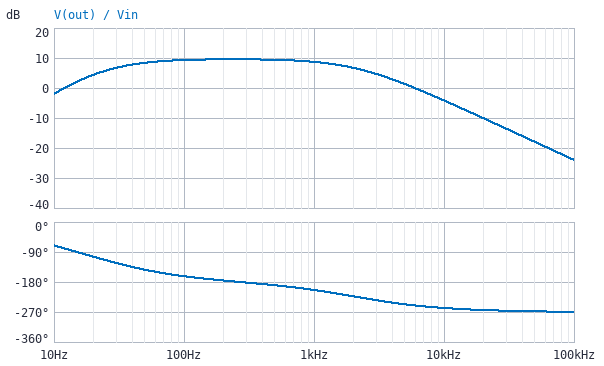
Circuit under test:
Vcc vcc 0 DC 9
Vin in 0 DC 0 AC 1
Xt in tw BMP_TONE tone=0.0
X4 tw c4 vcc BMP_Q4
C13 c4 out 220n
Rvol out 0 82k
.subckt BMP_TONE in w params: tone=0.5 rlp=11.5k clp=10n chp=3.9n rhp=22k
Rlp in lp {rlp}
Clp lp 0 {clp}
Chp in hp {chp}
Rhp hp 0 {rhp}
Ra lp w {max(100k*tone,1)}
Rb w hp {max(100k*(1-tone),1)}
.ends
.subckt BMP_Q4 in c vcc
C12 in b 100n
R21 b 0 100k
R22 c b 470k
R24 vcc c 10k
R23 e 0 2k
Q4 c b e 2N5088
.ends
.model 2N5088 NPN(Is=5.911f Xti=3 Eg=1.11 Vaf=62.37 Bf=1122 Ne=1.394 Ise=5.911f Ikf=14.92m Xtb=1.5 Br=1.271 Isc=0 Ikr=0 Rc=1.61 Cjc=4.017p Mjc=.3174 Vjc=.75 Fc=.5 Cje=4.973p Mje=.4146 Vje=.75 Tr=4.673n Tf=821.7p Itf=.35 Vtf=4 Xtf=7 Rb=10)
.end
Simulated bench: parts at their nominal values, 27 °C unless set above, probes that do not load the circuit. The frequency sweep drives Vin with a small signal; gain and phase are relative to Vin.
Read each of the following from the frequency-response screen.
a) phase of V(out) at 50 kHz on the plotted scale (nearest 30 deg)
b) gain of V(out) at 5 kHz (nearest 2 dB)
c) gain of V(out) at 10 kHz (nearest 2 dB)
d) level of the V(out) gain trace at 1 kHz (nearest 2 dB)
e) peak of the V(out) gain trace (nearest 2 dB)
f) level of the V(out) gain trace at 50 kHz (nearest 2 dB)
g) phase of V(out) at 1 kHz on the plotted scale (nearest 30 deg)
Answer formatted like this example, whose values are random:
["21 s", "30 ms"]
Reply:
["-270 deg", "2 dB", "-4 dB", "8 dB", "10 dB", "-18 dB", "-210 deg"]
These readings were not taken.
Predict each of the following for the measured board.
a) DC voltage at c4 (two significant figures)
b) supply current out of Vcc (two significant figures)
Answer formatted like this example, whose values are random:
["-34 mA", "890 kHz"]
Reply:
["6.5 V", "250 µA"]
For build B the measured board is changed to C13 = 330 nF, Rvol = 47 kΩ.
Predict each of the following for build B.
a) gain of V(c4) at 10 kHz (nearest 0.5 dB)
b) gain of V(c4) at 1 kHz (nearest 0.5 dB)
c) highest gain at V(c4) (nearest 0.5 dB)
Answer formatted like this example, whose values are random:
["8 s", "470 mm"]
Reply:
["-5.0 dB", "8.0 dB", "9.0 dB"]
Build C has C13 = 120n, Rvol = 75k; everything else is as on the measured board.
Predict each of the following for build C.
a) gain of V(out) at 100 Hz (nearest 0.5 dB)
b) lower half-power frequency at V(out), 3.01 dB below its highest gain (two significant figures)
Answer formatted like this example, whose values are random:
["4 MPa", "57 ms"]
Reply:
["9.0 dB", "33 Hz"]
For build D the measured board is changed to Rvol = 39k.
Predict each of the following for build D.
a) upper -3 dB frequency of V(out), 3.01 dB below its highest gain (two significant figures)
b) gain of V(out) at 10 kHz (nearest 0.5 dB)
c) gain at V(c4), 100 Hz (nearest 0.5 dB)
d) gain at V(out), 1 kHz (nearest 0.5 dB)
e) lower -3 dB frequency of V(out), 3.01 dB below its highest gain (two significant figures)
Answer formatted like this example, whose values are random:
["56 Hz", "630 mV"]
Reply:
["2.1 kHz", "-5.0 dB", "8.5 dB", "8.0 dB", "32 Hz"]
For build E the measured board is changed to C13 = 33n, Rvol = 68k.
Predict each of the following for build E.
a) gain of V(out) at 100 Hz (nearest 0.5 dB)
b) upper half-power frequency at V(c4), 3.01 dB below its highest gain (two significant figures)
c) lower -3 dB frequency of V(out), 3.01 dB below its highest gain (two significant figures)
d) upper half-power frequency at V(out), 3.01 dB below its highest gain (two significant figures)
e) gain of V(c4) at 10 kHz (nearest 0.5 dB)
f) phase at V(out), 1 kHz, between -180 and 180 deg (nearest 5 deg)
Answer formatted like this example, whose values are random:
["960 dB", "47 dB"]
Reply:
["8.0 dB", "2.0 kHz", "68 Hz", "2.2 kHz", "-4.5 dB", "160 deg"]
